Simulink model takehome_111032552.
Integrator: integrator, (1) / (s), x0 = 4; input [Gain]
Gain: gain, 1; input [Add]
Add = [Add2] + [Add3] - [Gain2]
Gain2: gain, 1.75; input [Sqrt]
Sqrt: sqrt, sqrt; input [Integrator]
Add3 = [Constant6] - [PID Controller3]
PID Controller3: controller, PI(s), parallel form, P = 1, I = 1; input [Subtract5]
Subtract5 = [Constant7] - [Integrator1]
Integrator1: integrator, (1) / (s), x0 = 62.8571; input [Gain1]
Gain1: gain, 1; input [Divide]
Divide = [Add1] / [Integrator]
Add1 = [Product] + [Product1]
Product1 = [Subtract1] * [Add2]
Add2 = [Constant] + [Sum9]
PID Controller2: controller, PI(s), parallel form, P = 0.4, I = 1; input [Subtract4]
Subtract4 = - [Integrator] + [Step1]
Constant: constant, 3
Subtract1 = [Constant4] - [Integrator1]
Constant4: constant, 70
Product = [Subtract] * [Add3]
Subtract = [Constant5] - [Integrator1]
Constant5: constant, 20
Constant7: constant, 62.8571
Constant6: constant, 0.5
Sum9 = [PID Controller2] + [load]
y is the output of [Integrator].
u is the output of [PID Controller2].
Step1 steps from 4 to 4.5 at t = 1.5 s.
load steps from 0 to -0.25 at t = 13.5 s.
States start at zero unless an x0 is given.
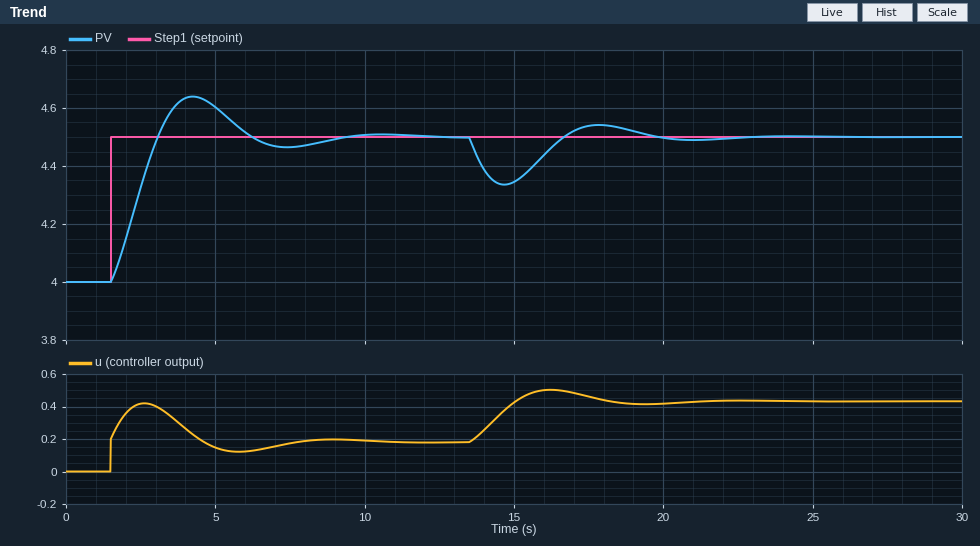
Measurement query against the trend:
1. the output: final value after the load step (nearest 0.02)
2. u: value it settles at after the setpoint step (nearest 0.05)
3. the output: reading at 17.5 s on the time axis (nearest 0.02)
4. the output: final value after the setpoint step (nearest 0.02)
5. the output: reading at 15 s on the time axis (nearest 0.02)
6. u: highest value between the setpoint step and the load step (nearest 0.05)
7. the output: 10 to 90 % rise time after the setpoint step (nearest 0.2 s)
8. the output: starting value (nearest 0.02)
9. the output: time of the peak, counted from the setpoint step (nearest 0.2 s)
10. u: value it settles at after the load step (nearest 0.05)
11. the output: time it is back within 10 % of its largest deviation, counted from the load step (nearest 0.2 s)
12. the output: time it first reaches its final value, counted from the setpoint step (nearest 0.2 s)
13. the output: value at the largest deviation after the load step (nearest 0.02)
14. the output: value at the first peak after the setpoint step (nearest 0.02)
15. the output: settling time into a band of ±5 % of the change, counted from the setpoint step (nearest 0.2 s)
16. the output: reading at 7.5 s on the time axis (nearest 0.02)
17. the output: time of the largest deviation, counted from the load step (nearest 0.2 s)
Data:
4.50
0.20
4.54
4.50
4.34
0.40
1.2 s
4.00
2.8 s
0.45
5.6 s
1.6 s
4.34
4.64
6.8 s
4.46
1.2 s
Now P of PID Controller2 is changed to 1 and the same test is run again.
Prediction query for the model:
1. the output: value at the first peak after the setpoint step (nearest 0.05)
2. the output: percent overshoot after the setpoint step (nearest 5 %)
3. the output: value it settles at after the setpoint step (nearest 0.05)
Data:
4.55
10 %
4.50
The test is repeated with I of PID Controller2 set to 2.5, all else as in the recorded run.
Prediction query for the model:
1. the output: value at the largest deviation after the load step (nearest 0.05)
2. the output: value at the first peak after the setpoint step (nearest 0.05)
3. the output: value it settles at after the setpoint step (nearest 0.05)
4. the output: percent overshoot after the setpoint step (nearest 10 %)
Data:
4.40
4.75
4.50
50 %
